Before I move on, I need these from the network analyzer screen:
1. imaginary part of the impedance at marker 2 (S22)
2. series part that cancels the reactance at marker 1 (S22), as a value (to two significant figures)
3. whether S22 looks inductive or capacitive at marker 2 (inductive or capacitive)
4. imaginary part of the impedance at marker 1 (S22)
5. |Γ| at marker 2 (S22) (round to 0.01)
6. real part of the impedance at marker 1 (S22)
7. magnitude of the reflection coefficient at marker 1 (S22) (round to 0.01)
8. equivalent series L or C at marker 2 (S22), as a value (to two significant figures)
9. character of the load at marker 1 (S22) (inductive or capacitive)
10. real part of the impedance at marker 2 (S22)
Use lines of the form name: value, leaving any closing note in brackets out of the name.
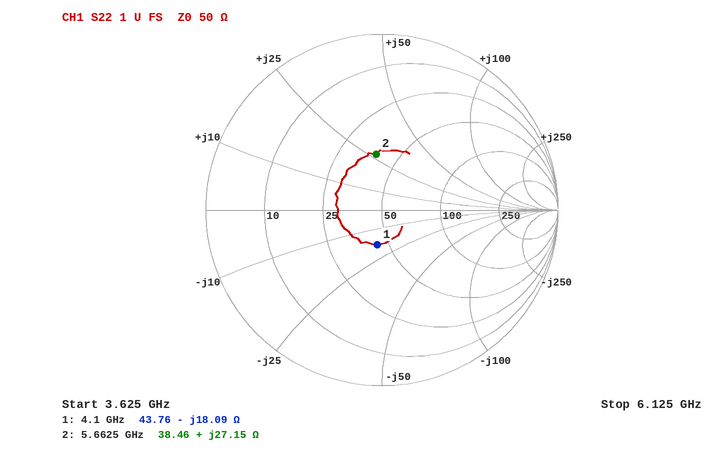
imaginary part of the impedance at marker 2: +27.15 Ω
series part that cancels the reactance at marker 1 (S22), as a value: 700 pH
whether S22 looks inductive or capacitive at marker 2: inductive
imaginary part of the impedance at marker 1: -18.09 Ω
|Γ| at marker 2 (S22): 0.32
real part of the impedance at marker 1: 43.76 Ω
magnitude of the reflection coefficient at marker 1 (S22): 0.20
equivalent series L or C at marker 2 (S22), as a value: 760 pH
character of the load at marker 1 (S22): capacitive
real part of the impedance at marker 2: 38.46 Ω
